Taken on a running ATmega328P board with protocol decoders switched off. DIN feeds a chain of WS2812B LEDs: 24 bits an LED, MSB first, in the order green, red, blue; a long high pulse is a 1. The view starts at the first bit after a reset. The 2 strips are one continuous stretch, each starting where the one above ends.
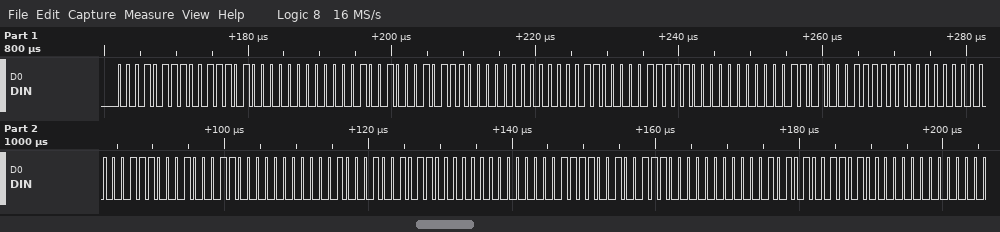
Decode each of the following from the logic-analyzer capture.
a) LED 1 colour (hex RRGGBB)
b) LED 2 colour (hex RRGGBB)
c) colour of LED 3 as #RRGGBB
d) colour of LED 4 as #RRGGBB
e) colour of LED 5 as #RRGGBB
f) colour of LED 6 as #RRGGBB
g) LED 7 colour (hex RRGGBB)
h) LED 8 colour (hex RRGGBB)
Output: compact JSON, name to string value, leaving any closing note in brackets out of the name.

{"LED 1 colour": "#3A1700", "LED 2 colour": "#2E1200", "colour of LED 3 as #RRGGBB": "#1F0C00", "colour of LED 4 as #RRGGBB": "#3F1A00", "colour of LED 5 as #RRGGBB": "#230E00", "colour of LED 6 as #RRGGBB": "#2C1100", "LED 7 colour": "#270F00", "LED 8 colour": "#341500"}
